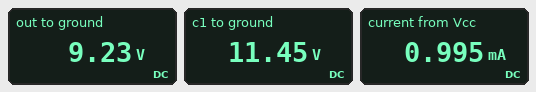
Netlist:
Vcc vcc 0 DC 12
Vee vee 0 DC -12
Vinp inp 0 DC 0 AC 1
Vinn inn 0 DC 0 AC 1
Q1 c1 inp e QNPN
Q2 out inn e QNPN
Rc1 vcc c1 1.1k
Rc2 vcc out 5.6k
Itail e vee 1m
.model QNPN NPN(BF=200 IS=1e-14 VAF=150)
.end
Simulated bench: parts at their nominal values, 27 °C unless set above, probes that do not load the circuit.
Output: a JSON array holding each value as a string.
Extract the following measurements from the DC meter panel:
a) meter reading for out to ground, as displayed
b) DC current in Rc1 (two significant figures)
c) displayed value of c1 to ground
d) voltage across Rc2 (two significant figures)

["9.23 V", "500 µA", "11.45 V", "2.8 V"]
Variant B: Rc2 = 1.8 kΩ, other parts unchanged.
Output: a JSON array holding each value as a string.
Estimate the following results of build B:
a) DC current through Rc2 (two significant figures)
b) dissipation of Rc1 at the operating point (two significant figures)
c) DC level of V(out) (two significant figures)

["500 µA", "270 µW", "11 V"]
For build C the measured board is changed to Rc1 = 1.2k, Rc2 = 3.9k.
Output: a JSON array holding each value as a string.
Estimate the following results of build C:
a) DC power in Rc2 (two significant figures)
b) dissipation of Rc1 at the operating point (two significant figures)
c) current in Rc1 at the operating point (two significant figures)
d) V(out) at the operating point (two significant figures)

["960 µW", "300 µW", "500 µA", "10 V"]
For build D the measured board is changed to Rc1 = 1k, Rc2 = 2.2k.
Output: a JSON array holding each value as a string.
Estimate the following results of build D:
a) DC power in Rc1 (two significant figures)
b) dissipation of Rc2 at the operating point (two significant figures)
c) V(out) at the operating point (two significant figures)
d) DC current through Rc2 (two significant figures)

["250 µW", "540 µW", "11 V", "500 µA"]
